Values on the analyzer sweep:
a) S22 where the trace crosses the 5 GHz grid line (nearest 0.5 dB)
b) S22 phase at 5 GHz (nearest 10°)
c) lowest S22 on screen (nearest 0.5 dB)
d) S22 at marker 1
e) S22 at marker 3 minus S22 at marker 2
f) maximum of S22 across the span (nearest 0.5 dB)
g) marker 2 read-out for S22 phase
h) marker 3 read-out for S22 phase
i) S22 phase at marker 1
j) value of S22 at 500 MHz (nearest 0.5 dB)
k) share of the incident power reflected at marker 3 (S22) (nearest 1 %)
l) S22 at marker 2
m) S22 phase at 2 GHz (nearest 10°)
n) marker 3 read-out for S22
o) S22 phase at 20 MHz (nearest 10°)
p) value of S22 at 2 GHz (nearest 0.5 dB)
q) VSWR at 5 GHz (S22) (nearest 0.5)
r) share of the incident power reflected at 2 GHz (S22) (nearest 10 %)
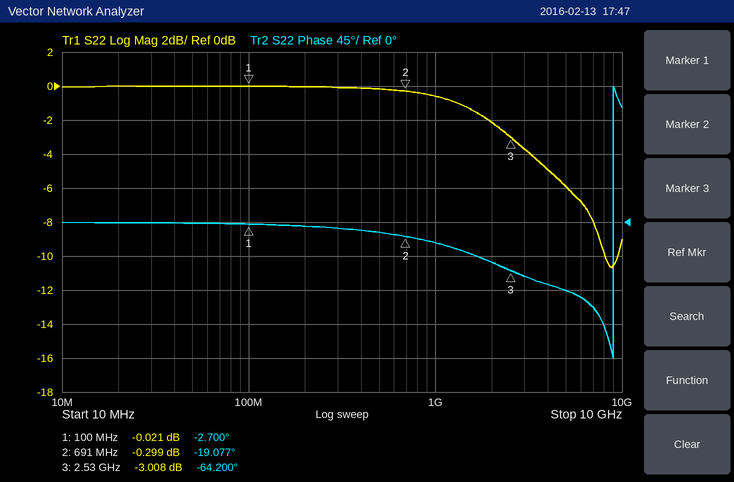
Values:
-6.0 dB
-90°
-10.5 dB
-0.021 dB
-2.709 dB
0.0 dB
-19.077°
-64.200°
-2.700°
0.0 dB
50 %
-0.299 dB
-50°
-3.008 dB
0°
-2.0 dB
3.0
60 %
